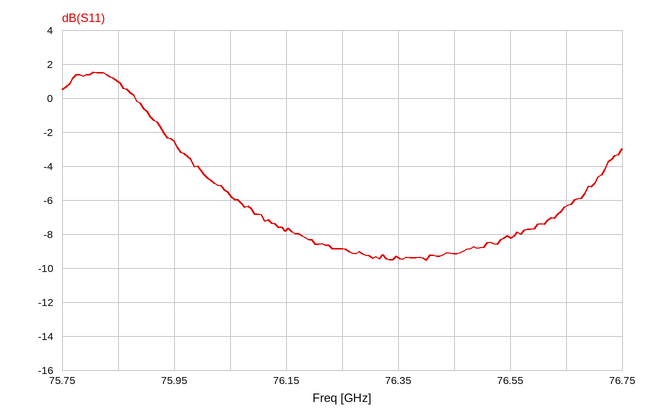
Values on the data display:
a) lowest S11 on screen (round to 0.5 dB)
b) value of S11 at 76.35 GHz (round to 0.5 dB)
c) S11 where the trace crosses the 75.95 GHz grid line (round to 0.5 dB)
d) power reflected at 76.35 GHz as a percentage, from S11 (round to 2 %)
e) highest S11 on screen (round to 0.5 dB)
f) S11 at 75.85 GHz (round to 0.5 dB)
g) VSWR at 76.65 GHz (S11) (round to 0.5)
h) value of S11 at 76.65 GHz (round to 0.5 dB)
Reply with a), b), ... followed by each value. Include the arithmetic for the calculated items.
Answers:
a) -9.5 dB
b) -9.5 dB
c) -2.5 dB
d) 10^(-9.5/10) ≈ 11.2 %, so 12 % to the nearest 2 %
e) 1.5 dB
f) 1.0 dB
g) |Γ| = 10^(-6.5/20) = 0.4732; VSWR = (1 + 0.4732)/(1 − 0.4732) ≈ 2.80, so 3.0 to the nearest 0.5
h) -6.5 dB
